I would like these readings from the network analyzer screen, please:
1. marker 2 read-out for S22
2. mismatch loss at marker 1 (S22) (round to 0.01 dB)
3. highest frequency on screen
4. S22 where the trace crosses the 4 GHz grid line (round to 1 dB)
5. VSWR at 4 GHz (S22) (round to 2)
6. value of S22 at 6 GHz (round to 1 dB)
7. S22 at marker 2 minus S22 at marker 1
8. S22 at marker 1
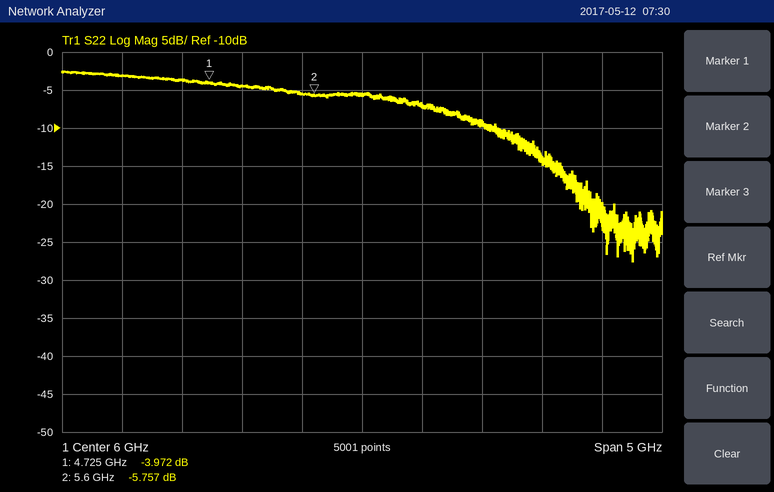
-5.757 dB
2.22 dB
8.5 GHz
-3 dB
6
-6 dB
-1.785 dB
-3.972 dB
